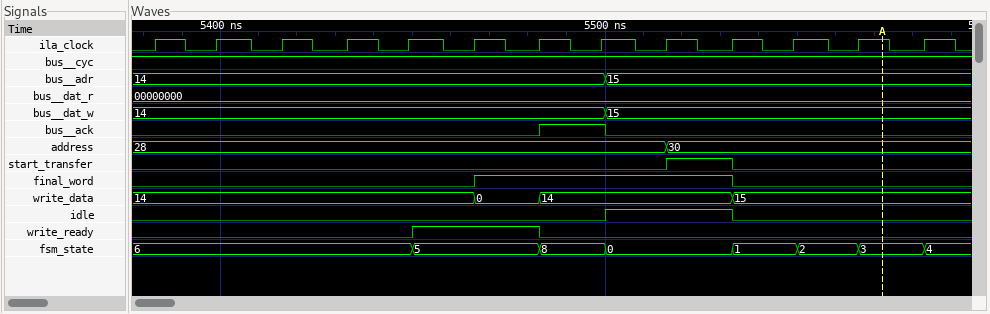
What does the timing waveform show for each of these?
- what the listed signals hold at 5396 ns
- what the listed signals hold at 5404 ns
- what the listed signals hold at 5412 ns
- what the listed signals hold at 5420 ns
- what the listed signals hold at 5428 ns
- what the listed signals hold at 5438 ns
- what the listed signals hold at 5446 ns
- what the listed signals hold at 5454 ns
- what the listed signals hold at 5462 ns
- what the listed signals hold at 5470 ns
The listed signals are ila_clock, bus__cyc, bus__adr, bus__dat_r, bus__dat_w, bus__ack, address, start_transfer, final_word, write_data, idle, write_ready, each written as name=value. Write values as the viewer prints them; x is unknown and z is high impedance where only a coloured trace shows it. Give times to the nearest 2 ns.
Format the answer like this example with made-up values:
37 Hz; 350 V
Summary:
ila_clock=0, bus__cyc=1, bus__adr=14, bus__dat_r=00000000, bus__dat_w=14, bus__ack=0, address=28, start_transfer=0, final_word=0, write_data=14, idle=0, write_ready=0; ila_clock=1, bus__cyc=1, bus__adr=14, bus__dat_r=00000000, bus__dat_w=14, bus__ack=0, address=28, start_transfer=0, final_word=0, write_data=14, idle=0, write_ready=0; ila_clock=0, bus__cyc=1, bus__adr=14, bus__dat_r=00000000, bus__dat_w=14, bus__ack=0, address=28, start_transfer=0, final_word=0, write_data=14, idle=0, write_ready=0; ila_clock=1, bus__cyc=1, bus__adr=14, bus__dat_r=00000000, bus__dat_w=14, bus__ack=0, address=28, start_transfer=0, final_word=0, write_data=14, idle=0, write_ready=0; ila_clock=0, bus__cyc=1, bus__adr=14, bus__dat_r=00000000, bus__dat_w=14, bus__ack=0, address=28, start_transfer=0, final_word=0, write_data=14, idle=0, write_ready=0; ila_clock=1, bus__cyc=1, bus__adr=14, bus__dat_r=00000000, bus__dat_w=14, bus__ack=0, address=28, start_transfer=0, final_word=0, write_data=14, idle=0, write_ready=0; ila_clock=0, bus__cyc=1, bus__adr=14, bus__dat_r=00000000, bus__dat_w=14, bus__ack=0, address=28, start_transfer=0, final_word=0, write_data=14, idle=0, write_ready=0; ila_clock=1, bus__cyc=1, bus__adr=14, bus__dat_r=00000000, bus__dat_w=14, bus__ack=0, address=28, start_transfer=0, final_word=0, write_data=14, idle=0, write_ready=1; ila_clock=0, bus__cyc=1, bus__adr=14, bus__dat_r=00000000, bus__dat_w=14, bus__ack=0, address=28, start_transfer=0, final_word=0, write_data=14, idle=0, write_ready=1; ila_clock=1, bus__cyc=1, bus__adr=14, bus__dat_r=00000000, bus__dat_w=14, bus__ack=0, address=28, start_transfer=0, final_word=1, write_data=0, idle=0, write_ready=1
